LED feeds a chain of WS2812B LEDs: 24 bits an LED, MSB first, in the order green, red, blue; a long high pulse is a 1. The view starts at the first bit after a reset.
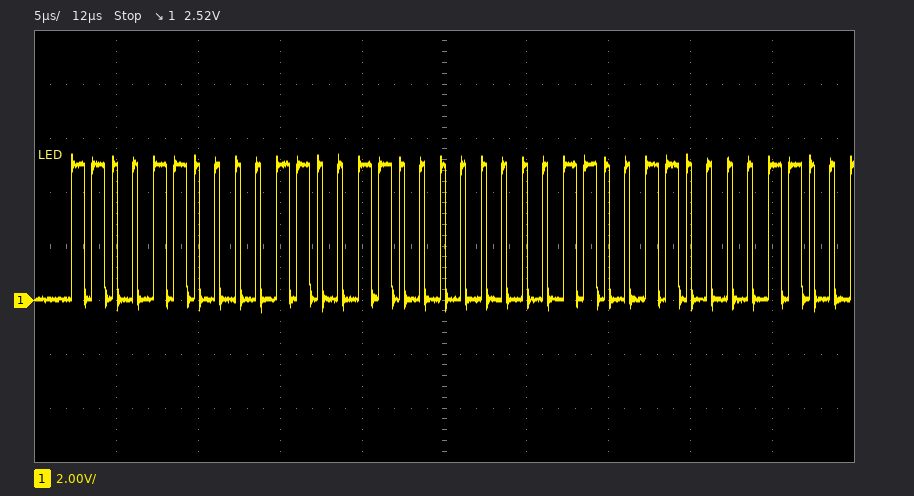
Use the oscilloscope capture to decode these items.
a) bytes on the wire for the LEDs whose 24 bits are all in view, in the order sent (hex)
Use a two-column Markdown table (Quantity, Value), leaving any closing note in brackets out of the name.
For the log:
| Quantity | Value |
|---|---|
| bytes on the wire for the LEDs whose 24 bits are all in view, in the order sent | CC 33 00 |
